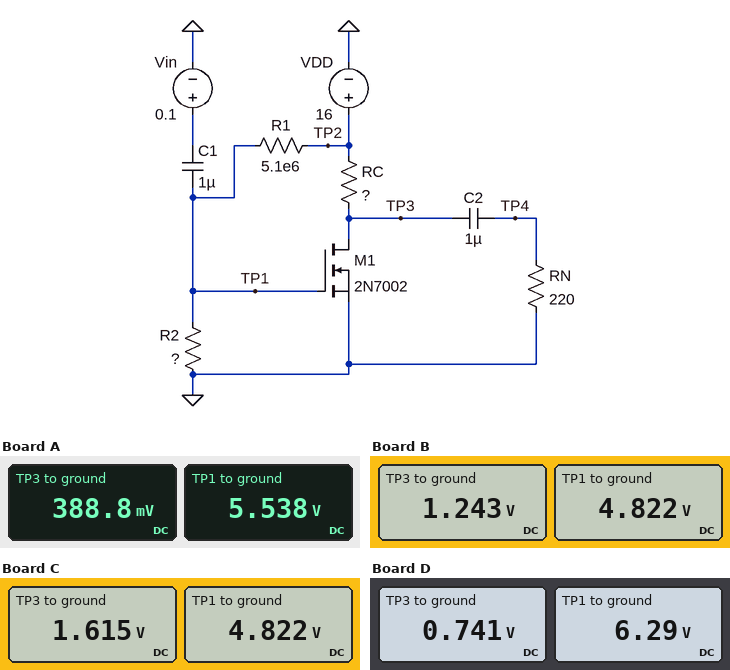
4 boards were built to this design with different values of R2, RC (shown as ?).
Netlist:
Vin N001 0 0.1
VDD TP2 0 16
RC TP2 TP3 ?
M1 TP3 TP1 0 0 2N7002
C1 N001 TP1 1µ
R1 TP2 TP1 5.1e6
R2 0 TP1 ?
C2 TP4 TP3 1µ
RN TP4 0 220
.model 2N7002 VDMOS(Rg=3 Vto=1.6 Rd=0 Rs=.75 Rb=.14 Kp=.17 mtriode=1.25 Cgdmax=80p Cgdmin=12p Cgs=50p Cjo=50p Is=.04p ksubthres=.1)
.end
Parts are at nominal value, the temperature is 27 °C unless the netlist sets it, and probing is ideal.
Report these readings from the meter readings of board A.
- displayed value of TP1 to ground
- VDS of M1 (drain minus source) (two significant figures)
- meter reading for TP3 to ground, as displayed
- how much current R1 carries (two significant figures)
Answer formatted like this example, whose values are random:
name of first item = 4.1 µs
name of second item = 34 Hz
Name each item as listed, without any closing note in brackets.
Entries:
displayed value of TP1 to ground = 5.538 V
VDS of M1 (drain minus source) = 390 mV
meter reading for TP3 to ground, as displayed = 388.8 mV
how much current R1 carries = 2.1 µA
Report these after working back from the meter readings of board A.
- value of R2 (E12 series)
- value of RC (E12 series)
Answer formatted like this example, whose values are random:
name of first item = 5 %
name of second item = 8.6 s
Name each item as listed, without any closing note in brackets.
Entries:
value of R2 = 2.7 MΩ
value of RC = 82 Ω
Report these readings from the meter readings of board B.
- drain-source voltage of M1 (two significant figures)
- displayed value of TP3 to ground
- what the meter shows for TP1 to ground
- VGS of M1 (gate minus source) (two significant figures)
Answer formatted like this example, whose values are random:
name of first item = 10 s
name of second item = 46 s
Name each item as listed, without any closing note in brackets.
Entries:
drain-source voltage of M1 = 1.2 V
displayed value of TP3 to ground = 1.243 V
what the meter shows for TP1 to ground = 4.822 V
VGS of M1 (gate minus source) = 4.8 V
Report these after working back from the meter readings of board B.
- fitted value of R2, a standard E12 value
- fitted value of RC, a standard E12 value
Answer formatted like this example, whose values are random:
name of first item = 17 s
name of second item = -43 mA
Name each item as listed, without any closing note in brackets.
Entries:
fitted value of R2, a standard E12 value = 2.2 MΩ
fitted value of RC, a standard E12 value = 33 Ω
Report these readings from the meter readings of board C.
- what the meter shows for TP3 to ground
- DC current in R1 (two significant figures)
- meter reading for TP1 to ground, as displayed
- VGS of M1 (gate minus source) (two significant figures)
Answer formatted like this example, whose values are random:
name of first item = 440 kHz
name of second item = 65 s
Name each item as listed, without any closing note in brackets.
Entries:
what the meter shows for TP3 to ground = 1.615 V
DC current in R1 = 2.2 µA
meter reading for TP1 to ground, as displayed = 4.822 V
VGS of M1 (gate minus source) = 4.8 V
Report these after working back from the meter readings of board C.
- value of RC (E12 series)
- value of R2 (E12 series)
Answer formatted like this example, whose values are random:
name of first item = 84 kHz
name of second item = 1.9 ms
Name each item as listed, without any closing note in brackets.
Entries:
value of RC = 27 Ω
value of R2 = 2.2 MΩ
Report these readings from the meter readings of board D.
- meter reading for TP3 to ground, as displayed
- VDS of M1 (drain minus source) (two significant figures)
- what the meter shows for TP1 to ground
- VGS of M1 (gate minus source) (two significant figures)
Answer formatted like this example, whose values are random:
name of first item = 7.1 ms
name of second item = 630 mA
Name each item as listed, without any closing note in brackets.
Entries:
meter reading for TP3 to ground, as displayed = 0.741 V
VDS of M1 (drain minus source) = 740 mV
what the meter shows for TP1 to ground = 6.29 V
VGS of M1 (gate minus source) = 6.3 V
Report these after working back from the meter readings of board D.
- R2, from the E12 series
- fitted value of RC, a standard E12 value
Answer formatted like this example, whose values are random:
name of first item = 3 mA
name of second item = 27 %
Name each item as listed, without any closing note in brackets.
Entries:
R2, from the E12 series = 3.3 MΩ
fitted value of RC, a standard E12 value = 39 Ω
